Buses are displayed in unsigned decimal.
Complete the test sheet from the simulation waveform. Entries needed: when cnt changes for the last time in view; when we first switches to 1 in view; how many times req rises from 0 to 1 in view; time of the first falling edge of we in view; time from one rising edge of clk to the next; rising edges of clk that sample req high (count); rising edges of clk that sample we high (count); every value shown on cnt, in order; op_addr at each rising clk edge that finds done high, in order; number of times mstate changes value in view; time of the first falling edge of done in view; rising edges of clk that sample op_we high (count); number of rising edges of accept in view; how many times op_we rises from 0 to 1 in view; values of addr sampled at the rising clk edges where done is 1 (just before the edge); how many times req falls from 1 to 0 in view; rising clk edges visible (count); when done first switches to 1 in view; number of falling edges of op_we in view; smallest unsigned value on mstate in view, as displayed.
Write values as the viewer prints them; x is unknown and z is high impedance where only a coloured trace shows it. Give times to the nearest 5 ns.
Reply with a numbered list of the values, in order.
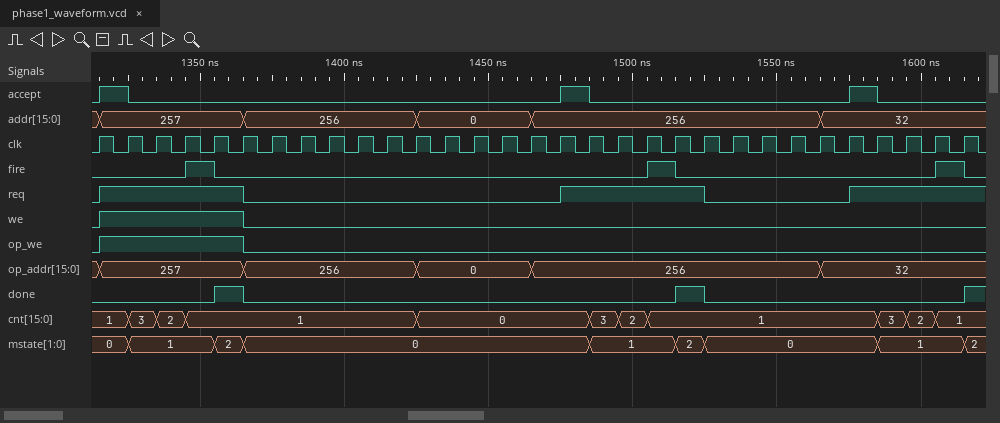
1. 1605 ns
2. 1315 ns
3. 3
4. 1365 ns
5. 10 ns
6. 14
7. 5
8. 1, 3, 2, 1, 0, 3, 2, 1, 3, 2, 1
9. 257, 256
10. 8
11. 1365 ns
12. 5
13. 3
14. 1
15. 257, 256
16. 2
17. 31
18. 1355 ns
19. 1
20. 0
